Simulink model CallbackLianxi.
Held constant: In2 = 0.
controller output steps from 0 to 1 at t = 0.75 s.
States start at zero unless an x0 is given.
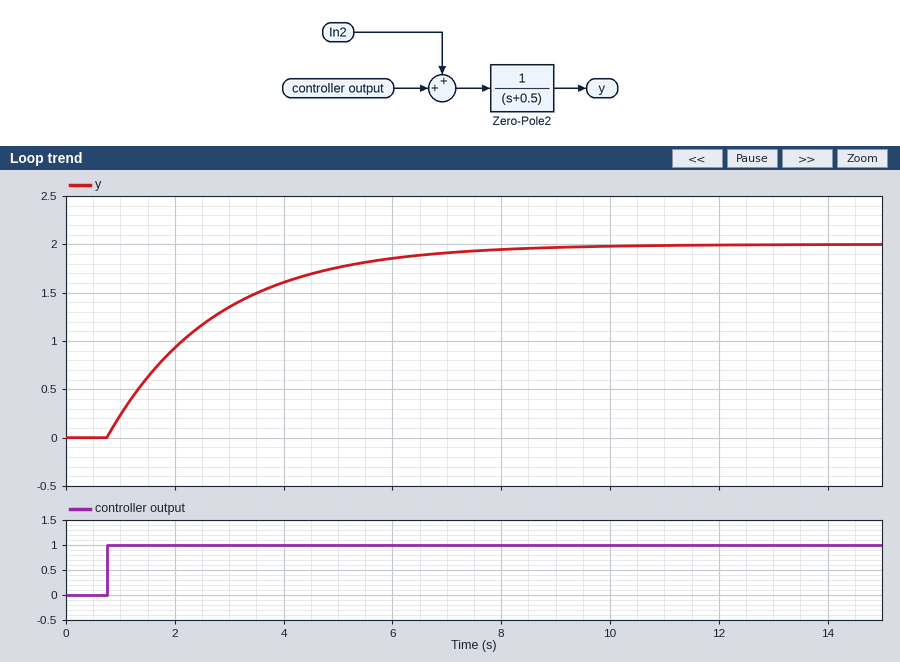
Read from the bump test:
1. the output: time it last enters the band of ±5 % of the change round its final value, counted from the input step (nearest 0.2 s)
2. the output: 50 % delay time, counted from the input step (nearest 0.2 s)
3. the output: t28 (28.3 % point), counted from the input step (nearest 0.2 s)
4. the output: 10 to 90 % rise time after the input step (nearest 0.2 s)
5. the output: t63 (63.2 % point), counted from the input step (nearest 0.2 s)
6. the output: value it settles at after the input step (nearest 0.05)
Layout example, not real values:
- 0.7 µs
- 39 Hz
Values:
- 6.0 s
- 1.4 s
- 0.6 s
- 4.4 s
- 2.0 s
- 2.00
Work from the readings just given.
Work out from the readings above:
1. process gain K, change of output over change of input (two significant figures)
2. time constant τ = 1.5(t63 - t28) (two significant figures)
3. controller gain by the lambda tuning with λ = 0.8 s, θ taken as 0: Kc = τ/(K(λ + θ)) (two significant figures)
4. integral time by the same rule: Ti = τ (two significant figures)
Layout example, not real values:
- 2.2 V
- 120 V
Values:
- 2.0
- 2.1 s
- 1.3
- 2.1 s
